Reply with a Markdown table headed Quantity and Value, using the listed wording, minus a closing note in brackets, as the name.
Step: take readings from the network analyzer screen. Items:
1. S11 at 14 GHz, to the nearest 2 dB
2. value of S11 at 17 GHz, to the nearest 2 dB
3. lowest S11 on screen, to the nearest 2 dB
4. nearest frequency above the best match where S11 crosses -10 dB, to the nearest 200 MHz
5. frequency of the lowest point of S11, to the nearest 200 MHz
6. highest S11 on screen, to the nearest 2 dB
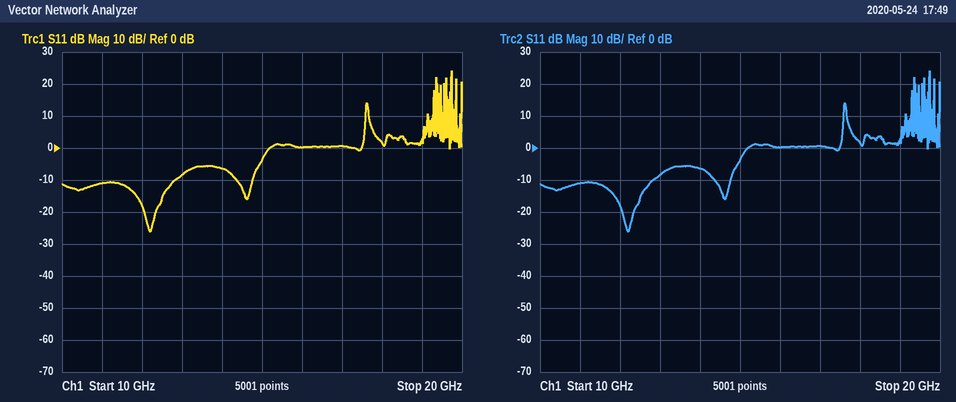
| Quantity | Value |
|---|---|
| S11 at 14 GHz, to the nearest 2 dB | -6 dB |
| value of S11 at 17 GHz, to the nearest 2 dB | 0 dB |
| lowest S11 on screen, to the nearest 2 dB | -26 dB |
| nearest frequency above the best match where S11 crosses -10 dB, to the nearest 200 MHz | 12.8 GHz |
| frequency of the lowest point of S11, to the nearest 200 MHz | 12.2 GHz |
| highest S11 on screen, to the nearest 2 dB | 24 dB |
